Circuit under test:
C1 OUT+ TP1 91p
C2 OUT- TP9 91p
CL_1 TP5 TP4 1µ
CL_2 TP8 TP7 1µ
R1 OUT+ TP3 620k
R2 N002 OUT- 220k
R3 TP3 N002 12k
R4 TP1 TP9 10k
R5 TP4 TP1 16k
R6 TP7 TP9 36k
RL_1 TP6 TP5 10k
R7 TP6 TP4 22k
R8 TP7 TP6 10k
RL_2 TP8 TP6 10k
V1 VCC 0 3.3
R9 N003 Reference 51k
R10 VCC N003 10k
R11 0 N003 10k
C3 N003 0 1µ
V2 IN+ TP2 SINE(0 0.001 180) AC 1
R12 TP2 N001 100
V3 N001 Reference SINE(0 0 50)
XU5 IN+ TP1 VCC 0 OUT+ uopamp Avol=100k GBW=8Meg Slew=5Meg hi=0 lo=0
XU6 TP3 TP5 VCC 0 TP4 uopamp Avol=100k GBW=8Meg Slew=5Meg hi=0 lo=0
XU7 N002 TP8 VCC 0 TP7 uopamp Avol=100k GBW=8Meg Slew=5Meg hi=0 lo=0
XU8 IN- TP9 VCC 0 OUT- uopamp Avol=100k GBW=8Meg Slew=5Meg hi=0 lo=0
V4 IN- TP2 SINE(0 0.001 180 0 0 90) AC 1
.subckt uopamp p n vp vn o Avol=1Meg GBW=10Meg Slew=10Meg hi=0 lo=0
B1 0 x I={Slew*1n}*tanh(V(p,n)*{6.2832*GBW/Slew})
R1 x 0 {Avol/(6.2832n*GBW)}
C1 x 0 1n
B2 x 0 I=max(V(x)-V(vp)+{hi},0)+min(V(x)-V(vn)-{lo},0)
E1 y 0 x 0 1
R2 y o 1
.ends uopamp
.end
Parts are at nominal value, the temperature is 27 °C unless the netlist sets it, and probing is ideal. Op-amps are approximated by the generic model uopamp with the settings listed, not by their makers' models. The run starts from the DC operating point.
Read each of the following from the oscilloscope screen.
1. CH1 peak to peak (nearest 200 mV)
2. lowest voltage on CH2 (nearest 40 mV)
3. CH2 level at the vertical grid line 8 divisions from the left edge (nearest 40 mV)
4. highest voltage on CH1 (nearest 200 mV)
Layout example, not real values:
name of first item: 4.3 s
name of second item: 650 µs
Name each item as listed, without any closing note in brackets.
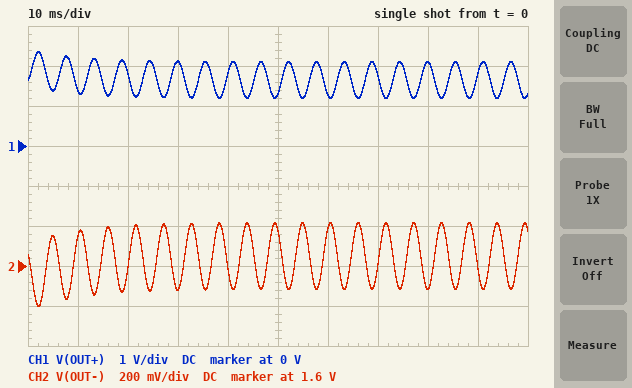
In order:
CH1 peak to peak: 1.2 V
lowest voltage on CH2: 1.40 V
CH2 level at the vertical grid line 8 divisions from the left edge: 1.48 V
highest voltage on CH1: 2.4 V
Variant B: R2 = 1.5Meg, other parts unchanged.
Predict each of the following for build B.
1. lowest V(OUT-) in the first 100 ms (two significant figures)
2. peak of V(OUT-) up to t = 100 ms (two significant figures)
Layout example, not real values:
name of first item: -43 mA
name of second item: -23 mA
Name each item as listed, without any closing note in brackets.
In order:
lowest V(OUT-) in the first 100 ms: 69 mV
peak of V(OUT-) up to t = 100 ms: 2.6 V
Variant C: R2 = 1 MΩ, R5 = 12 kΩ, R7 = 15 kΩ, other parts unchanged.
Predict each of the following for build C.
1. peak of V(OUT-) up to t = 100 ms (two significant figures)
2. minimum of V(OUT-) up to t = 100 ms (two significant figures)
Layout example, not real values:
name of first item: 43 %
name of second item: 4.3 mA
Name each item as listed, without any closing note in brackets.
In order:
peak of V(OUT-) up to t = 100 ms: 2.3 V
minimum of V(OUT-) up to t = 100 ms: 630 mV
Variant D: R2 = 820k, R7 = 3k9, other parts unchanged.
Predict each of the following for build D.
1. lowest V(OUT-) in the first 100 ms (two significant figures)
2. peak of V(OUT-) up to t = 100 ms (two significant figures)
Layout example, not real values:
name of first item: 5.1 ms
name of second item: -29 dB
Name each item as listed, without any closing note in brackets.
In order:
lowest V(OUT-) in the first 100 ms: 750 mV
peak of V(OUT-) up to t = 100 ms: 2.2 V
